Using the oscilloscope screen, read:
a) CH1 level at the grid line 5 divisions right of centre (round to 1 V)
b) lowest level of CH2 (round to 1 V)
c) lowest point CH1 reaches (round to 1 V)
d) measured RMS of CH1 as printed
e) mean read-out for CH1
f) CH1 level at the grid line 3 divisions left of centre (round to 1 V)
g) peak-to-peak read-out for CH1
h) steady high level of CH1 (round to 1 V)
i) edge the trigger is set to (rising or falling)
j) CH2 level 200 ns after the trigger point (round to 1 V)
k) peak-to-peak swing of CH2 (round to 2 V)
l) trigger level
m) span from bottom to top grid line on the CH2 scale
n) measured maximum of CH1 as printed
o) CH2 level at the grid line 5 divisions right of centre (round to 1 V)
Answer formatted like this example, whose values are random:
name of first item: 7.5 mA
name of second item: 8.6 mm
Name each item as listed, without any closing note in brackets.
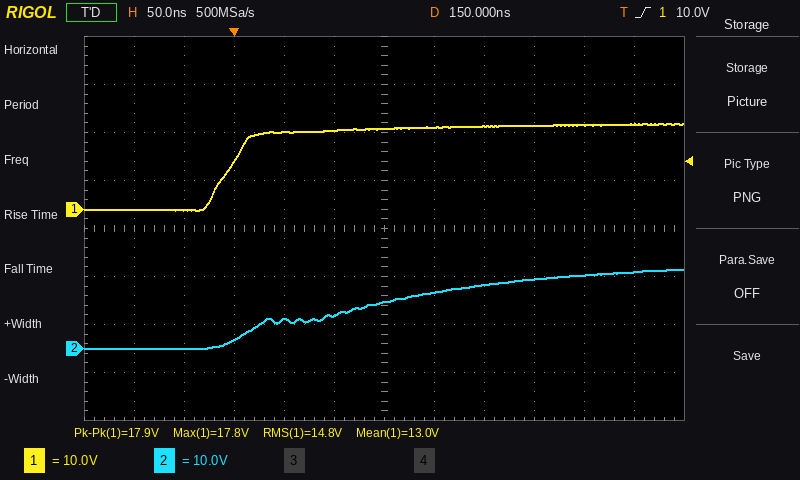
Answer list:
CH1 level at the grid line 5 divisions right of centre: 18 V
lowest level of CH2: 0 V
lowest point CH1 reaches: 0 V
measured RMS of CH1 as printed: 14.8 V
mean read-out for CH1: 13.0 V
CH1 level at the grid line 3 divisions left of centre: 10 V
peak-to-peak read-out for CH1: 17.9 V
steady high level of CH1: 17 V
edge the trigger is set to: rising
CH2 level 200 ns after the trigger point: 12 V
peak-to-peak swing of CH2: 16 V
trigger level: 10.0 V
span from bottom to top grid line on the CH2 scale: 80 V
measured maximum of CH1 as printed: 17.8 V
CH2 level at the grid line 5 divisions right of centre: 16 V
